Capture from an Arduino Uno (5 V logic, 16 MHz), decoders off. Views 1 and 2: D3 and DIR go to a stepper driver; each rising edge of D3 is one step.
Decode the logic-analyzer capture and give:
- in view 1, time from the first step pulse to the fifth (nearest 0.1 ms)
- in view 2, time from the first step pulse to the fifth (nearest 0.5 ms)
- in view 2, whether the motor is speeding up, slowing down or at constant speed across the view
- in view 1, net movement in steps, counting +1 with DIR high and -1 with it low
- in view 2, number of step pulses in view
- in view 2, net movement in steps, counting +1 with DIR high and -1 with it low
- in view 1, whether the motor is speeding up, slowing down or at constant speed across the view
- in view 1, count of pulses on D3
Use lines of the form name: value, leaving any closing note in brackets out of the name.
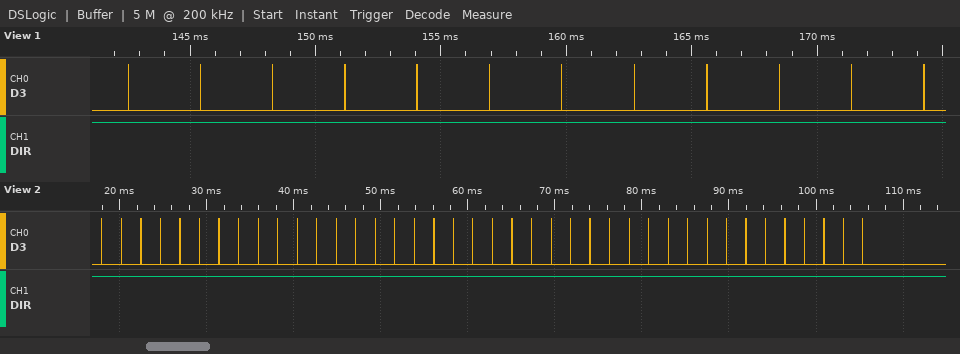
in view 1, time from the first step pulse to the fifth: 11.5 ms
in view 2, time from the first step pulse to the fifth: 9.0 ms
in view 2, whether the motor is speeding up, slowing down or at constant speed across the view: constant speed
in view 1, net movement in steps, counting +1 with DIR high and -1 with it low: +12
in view 2, number of step pulses in view: 40
in view 2, net movement in steps, counting +1 with DIR high and -1 with it low: +40
in view 1, whether the motor is speeding up, slowing down or at constant speed across the view: constant speed
in view 1, count of pulses on D3: 12
